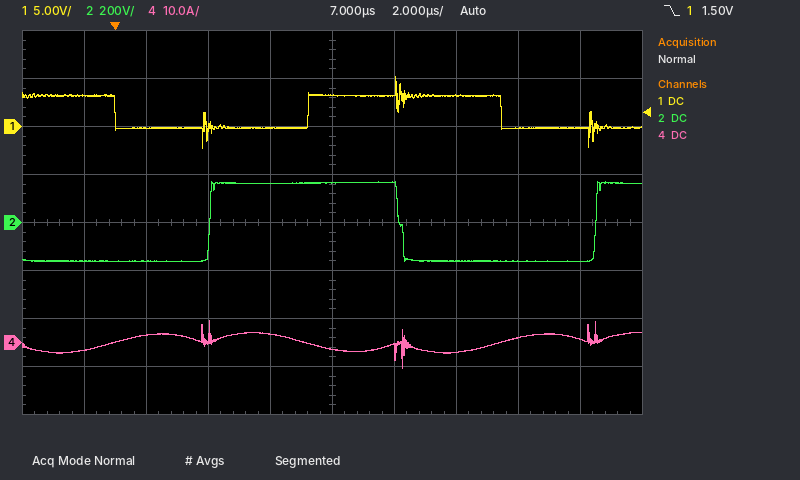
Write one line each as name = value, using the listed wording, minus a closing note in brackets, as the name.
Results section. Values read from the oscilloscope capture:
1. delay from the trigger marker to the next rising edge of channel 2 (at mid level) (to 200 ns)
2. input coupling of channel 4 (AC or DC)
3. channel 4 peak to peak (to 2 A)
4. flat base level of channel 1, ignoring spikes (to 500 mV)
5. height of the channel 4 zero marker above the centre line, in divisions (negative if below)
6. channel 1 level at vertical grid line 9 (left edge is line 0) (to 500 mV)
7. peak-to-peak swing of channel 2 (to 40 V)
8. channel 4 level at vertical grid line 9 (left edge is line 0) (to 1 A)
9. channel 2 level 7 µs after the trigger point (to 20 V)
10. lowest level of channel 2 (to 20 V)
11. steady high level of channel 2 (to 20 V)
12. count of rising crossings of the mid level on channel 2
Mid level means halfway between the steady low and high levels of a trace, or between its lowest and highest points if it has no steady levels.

delay from the trigger marker to the next rising edge of channel 2 (at mid level) = 3.0 µs
input coupling of channel 4 = DC
channel 4 peak to peak = 10 A
flat base level of channel 1, ignoring spikes = 0.0 V
height of the channel 4 zero marker above the centre line, in divisions = -2.5 div
channel 1 level at vertical grid line 9 (left edge is line 0) = 0.0 V
peak-to-peak swing of channel 2 = 320 V
channel 4 level at vertical grid line 9 (left edge is line 0) = 1 A
channel 2 level 7 µs after the trigger point = 160 V
lowest level of channel 2 = -160 V
steady high level of channel 2 = 160 V
count of rising crossings of the mid level on channel 2 = 2
